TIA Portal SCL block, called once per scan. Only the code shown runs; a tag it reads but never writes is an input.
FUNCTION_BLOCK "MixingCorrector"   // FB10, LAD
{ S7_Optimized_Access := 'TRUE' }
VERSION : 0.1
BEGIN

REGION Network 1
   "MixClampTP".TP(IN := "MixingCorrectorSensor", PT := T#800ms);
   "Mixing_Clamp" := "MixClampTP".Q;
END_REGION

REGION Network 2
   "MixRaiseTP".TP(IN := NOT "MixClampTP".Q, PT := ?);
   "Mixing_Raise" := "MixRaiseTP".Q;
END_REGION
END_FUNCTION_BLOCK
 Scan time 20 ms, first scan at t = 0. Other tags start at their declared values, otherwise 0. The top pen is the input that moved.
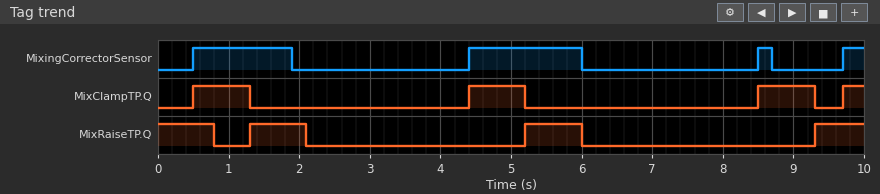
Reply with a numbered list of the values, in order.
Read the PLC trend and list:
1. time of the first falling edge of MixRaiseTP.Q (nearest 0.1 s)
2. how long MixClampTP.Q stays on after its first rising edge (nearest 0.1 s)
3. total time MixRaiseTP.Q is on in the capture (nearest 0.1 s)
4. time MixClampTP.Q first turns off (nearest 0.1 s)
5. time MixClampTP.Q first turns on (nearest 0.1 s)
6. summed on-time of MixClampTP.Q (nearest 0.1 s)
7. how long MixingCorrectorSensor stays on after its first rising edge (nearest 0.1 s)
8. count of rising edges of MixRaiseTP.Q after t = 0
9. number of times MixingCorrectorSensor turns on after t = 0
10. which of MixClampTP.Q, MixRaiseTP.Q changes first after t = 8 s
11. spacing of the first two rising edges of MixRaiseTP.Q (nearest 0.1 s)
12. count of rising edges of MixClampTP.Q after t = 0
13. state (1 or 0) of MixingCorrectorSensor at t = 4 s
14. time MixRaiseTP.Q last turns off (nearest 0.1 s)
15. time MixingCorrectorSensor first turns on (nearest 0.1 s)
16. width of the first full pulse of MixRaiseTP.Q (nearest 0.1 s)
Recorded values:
1. 0.8 s
2. 0.8 s
3. 3.1 s
4. 1.3 s
5. 0.5 s
6. 2.7 s
7. 1.4 s
8. 3
9. 4
10. MixClampTP.Q
11. 3.9 s
12. 4
13. 0
14. 6.0 s
15. 0.5 s
16. 0.8 s
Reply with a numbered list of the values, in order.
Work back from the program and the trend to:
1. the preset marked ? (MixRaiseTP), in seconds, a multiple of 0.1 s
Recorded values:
1. 0.8 s
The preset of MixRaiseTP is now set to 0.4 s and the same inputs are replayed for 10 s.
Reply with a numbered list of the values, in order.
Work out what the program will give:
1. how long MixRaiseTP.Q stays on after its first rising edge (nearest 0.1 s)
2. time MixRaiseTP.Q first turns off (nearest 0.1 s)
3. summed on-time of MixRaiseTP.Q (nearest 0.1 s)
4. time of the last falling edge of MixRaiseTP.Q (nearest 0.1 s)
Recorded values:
1. 0.4 s
2. 0.4 s
3. 1.6 s
4. 9.7 s
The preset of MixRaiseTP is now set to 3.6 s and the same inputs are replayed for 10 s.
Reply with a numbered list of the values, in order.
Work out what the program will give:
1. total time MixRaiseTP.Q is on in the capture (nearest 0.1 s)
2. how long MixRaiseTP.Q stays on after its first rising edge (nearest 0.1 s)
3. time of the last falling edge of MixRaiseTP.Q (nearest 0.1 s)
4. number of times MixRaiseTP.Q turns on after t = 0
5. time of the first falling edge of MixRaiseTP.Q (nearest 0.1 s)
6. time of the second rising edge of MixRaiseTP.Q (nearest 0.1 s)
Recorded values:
1. 7.9 s
2. 3.6 s
3. 8.8 s
4. 2
5. 3.6 s
6. 9.3 s
